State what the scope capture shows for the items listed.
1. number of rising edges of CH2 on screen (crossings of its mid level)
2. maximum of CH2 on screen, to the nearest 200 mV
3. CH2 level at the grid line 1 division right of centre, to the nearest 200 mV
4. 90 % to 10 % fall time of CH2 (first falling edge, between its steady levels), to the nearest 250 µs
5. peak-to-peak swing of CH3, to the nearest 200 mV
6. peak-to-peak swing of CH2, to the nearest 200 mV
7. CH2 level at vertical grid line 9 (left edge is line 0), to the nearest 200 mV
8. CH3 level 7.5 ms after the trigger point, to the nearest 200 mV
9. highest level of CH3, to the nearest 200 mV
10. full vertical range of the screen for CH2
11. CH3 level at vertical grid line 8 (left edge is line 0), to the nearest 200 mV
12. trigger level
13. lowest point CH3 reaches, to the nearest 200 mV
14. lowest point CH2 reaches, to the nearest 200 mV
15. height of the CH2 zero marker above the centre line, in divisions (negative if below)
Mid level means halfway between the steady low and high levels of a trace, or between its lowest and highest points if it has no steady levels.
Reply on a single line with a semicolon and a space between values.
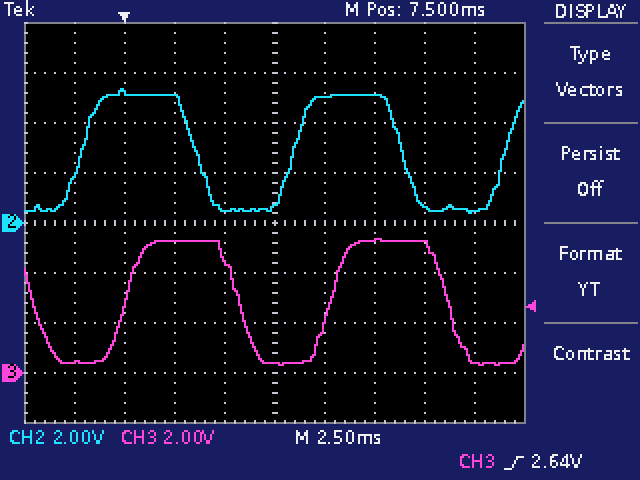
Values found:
3; 5.4 V; 5.0 V; 1.50 ms; 5.0 V; 5.0 V; 400 mV; 400 mV; 5.4 V; 16 V; 5.2 V; 2.64 V; 400 mV; 400 mV; 0.0 div
